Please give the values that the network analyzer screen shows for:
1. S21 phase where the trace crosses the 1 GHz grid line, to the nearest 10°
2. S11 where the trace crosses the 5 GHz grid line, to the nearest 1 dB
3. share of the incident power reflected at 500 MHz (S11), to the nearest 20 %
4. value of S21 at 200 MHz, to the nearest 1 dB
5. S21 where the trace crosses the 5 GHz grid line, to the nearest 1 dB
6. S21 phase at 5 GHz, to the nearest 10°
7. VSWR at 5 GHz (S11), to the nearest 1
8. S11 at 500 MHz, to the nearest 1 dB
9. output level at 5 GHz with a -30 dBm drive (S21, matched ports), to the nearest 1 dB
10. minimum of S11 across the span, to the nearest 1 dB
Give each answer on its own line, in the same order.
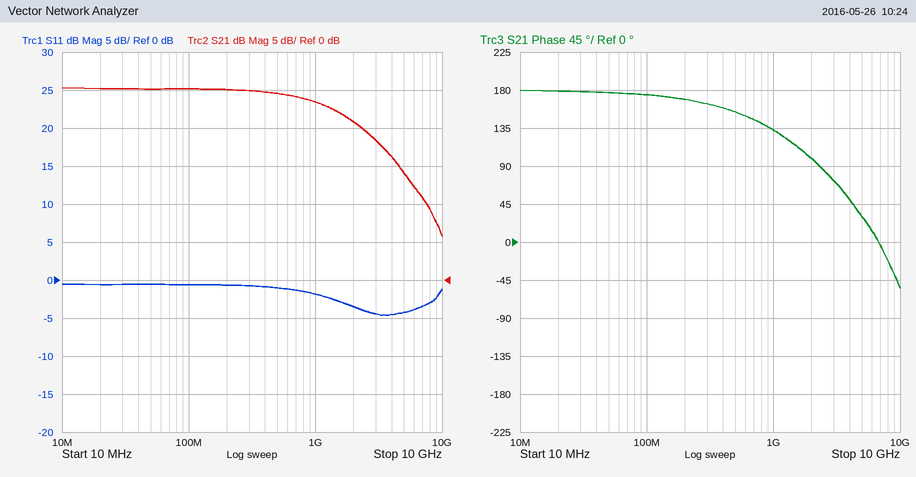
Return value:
130°
-4 dB
80 %
25 dB
14 dB
30°
4
-1 dB
-16 dBm
-5 dB
